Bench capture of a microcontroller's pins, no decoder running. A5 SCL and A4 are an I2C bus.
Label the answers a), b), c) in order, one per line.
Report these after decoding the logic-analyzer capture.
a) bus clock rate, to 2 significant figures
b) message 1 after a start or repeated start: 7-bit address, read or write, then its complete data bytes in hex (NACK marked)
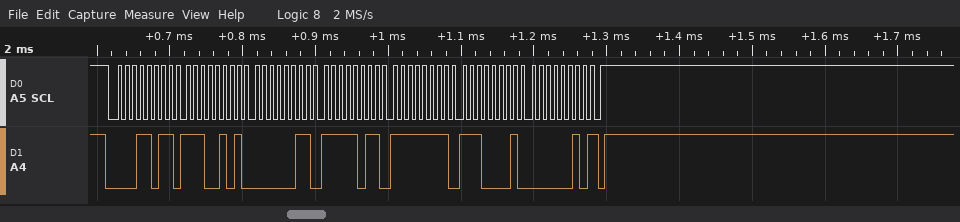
a) 100 kHz
b) 0x0D read: E5 03 FB FF E1 02 NACK
